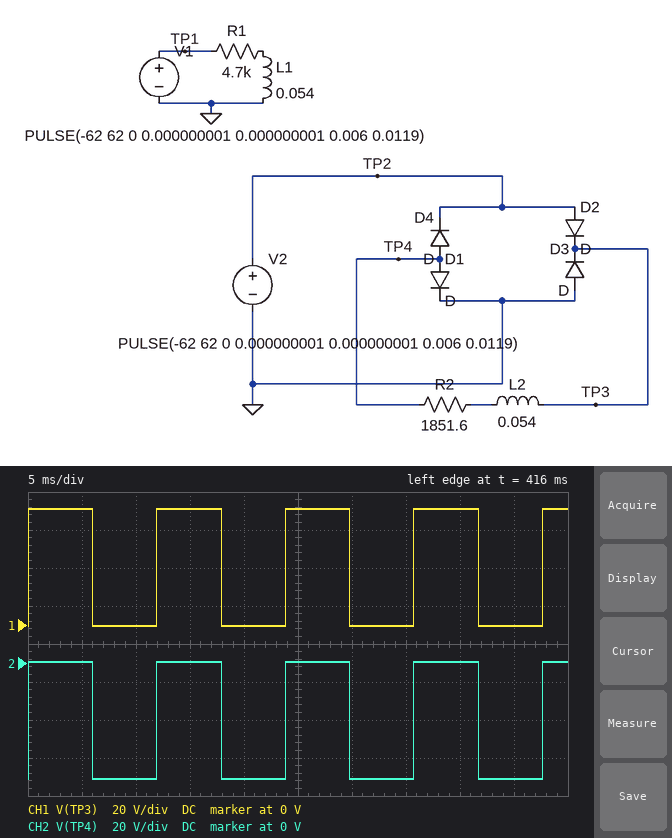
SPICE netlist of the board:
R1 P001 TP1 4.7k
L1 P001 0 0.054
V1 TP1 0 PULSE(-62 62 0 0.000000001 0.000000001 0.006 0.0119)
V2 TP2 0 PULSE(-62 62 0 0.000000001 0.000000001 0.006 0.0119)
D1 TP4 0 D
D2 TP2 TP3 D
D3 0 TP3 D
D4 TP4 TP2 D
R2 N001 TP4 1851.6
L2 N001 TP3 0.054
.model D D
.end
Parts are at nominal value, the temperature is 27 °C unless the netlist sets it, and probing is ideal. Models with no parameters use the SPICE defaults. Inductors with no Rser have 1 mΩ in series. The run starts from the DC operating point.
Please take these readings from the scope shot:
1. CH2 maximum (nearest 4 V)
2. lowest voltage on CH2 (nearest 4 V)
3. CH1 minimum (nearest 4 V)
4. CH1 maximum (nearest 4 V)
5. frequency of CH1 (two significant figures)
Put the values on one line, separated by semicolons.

0 V; -60 V; 0 V; 60 V; 84 Hz
